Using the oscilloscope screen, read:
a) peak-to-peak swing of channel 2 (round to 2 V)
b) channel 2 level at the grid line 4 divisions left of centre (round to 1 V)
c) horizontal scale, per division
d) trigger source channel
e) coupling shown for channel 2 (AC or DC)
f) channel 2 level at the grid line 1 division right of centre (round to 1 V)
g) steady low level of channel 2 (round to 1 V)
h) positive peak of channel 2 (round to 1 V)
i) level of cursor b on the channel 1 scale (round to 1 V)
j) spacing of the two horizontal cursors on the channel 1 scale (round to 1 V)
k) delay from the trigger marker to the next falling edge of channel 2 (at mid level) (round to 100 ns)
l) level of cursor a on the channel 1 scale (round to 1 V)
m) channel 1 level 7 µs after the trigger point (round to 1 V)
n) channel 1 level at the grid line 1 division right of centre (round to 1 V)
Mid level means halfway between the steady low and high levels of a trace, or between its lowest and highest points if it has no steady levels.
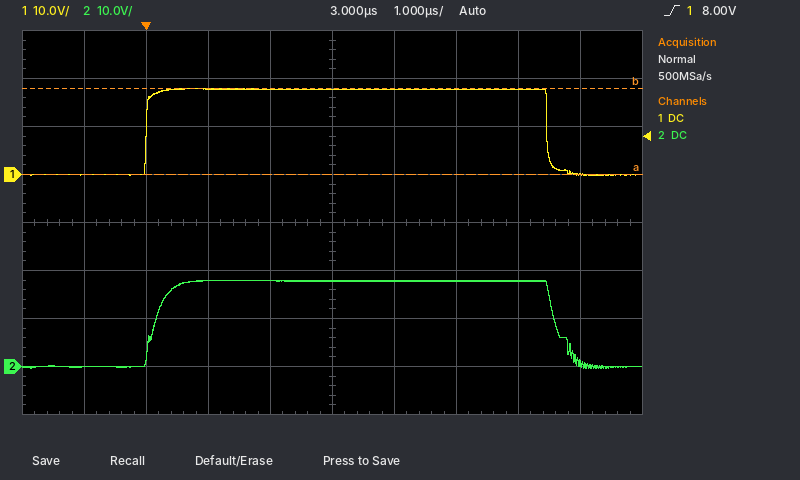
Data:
18 V
0 V
1 µs
channel 1
DC
18 V
0 V
18 V
18 V
18 V
6.6 µs
0 V
0 V
18 V
